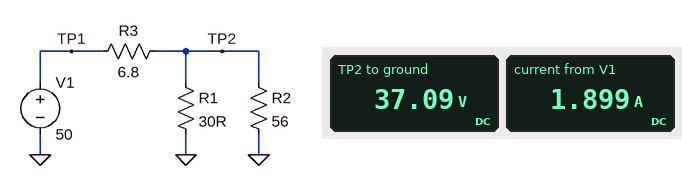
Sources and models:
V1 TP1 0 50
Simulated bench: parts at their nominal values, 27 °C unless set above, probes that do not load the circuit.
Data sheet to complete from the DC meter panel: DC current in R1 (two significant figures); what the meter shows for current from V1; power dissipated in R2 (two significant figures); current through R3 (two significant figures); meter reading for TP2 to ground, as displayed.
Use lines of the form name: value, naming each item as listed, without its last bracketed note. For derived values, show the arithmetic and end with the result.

DC current in R1: (37.09 V) / 30 Ω = 1.2 A
what the meter shows for current from V1: 1.899 A
power dissipated in R2: (37.09 V)^2 / 56 Ω = 25 W
current through R3: (50 V - 37.09 V) / 6.8 Ω = 1.9 A
meter reading for TP2 to ground, as displayed: 37.09 V
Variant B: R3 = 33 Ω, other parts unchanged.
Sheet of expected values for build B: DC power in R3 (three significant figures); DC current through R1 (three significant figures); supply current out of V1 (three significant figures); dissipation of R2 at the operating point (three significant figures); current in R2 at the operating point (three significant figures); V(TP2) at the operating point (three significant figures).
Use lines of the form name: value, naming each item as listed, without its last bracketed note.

DC power in R3: 29.9 W
DC current through R1: 620 mA
supply current out of V1: 952 mA
dissipation of R2 at the operating point: 6.17 W
current in R2 at the operating point: 332 mA
V(TP2) at the operating point: 18.6 V
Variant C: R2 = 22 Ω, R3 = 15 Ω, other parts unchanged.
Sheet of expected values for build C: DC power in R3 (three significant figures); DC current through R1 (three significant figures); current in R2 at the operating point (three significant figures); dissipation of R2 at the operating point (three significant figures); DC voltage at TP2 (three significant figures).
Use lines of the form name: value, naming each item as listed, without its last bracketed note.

DC power in R3: 48.9 W
DC current through R1: 764 mA
current in R2 at the operating point: 1.04 A
dissipation of R2 at the operating point: 23.9 W
DC voltage at TP2: 22.9 V
